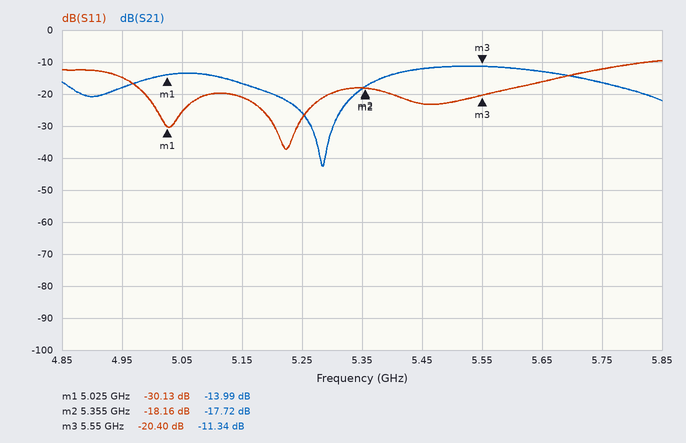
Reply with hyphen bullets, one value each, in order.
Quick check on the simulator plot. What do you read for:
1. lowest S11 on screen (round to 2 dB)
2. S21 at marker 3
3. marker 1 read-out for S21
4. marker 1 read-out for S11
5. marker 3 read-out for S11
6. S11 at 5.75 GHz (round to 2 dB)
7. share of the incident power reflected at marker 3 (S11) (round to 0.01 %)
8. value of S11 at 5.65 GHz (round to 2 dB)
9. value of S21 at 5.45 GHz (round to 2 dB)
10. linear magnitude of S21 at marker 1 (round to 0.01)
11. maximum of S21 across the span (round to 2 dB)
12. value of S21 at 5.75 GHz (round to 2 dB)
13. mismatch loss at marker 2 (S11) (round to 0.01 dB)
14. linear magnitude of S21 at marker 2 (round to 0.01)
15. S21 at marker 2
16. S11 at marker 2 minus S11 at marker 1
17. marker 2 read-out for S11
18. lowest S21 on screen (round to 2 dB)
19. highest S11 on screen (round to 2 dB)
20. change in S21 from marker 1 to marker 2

- -38 dB
- -11.34 dB
- -13.99 dB
- -30.13 dB
- -20.40 dB
- -12 dB
- 0.91 %
- -16 dB
- -12 dB
- 0.20
- -12 dB
- -16 dB
- 0.07 dB
- 0.13
- -17.72 dB
- 11.97 dB
- -18.16 dB
- -42 dB
- -10 dB
- -3.73 dB
